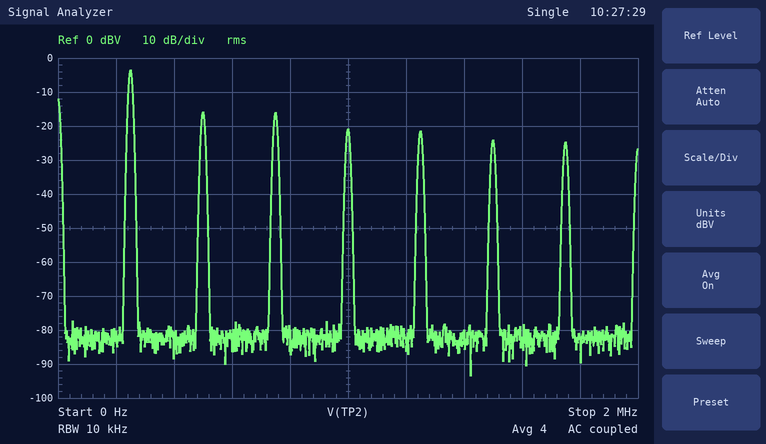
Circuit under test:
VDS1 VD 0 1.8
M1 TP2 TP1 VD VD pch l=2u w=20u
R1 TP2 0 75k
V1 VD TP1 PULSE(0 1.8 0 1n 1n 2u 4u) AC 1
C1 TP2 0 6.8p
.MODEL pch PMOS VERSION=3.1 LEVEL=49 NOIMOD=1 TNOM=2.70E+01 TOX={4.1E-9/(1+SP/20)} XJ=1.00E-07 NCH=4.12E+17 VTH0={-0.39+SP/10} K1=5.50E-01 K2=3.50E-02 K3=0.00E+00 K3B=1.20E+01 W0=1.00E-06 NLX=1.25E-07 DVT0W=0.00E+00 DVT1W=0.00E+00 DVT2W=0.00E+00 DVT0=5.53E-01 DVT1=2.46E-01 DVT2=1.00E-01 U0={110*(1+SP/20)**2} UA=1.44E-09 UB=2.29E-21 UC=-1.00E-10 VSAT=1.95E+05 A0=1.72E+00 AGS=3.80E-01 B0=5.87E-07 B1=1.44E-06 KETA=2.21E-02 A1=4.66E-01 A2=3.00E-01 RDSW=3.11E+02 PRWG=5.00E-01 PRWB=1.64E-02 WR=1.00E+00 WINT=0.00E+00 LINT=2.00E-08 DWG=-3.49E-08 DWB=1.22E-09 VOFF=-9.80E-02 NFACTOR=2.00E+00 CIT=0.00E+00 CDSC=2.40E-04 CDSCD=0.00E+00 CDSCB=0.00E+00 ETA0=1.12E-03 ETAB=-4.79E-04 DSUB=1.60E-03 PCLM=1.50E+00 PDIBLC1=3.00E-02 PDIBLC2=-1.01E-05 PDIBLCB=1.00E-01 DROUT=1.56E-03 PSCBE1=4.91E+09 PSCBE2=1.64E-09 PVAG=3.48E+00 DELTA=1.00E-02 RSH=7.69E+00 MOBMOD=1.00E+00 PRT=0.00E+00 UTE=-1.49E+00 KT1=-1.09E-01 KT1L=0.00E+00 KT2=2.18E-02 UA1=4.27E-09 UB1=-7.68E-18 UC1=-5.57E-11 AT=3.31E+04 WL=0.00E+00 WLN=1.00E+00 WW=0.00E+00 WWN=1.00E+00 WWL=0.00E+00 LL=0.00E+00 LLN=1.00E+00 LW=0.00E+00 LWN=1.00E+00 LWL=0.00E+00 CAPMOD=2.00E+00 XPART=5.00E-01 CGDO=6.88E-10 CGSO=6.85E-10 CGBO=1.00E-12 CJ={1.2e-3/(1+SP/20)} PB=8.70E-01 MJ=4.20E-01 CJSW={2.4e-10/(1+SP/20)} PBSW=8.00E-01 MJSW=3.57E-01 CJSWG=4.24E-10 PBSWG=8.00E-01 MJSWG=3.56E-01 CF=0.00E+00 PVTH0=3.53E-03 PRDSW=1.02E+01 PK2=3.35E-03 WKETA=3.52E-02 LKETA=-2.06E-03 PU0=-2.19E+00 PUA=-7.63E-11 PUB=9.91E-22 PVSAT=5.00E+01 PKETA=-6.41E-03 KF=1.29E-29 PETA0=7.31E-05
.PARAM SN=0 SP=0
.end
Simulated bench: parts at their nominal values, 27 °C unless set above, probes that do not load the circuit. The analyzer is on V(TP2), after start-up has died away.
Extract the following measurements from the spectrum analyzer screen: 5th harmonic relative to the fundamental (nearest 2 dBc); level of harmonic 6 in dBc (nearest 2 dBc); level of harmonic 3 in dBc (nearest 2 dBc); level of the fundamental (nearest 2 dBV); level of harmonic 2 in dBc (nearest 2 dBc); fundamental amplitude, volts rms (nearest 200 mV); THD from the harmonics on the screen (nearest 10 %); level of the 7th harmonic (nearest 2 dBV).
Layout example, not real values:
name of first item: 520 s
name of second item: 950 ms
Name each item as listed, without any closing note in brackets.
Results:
5th harmonic relative to the fundamental: -18 dBc
level of harmonic 6 in dBc: -20 dBc
level of harmonic 3 in dBc: -12 dBc
level of the fundamental: -4 dBV
level of harmonic 2 in dBc: -12 dBc
fundamental amplitude, volts rms: 600 mV
THD from the harmonics on the screen: 40 %
level of the 7th harmonic: -24 dBV
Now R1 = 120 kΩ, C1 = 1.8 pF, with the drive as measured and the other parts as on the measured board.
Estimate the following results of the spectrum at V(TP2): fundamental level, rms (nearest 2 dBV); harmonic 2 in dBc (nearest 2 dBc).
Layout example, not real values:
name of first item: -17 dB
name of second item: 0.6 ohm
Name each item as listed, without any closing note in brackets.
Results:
fundamental level, rms: -2 dBV
harmonic 2 in dBc: -16 dBc
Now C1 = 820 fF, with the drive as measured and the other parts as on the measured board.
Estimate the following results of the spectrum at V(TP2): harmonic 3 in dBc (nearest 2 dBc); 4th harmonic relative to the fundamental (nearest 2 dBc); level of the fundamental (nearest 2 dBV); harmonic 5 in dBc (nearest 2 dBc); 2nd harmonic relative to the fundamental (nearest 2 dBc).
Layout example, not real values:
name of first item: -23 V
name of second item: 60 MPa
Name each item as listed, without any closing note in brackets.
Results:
harmonic 3 in dBc: -10 dBc
4th harmonic relative to the fundamental: -26 dBc
level of the fundamental: -2 dBV
harmonic 5 in dBc: -14 dBc
2nd harmonic relative to the fundamental: -26 dBc
